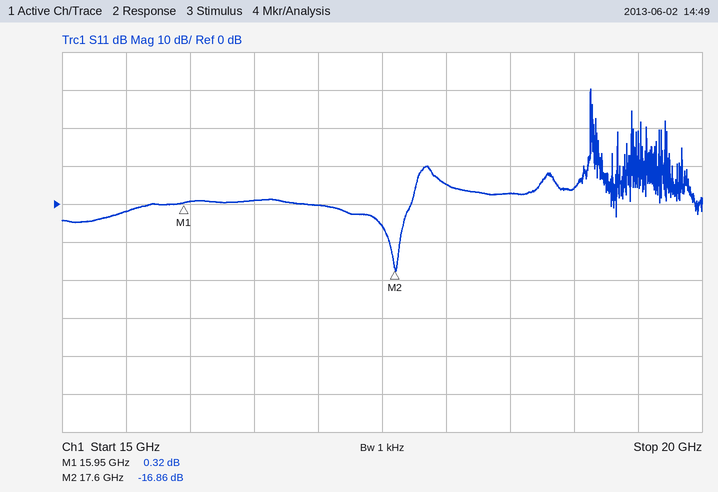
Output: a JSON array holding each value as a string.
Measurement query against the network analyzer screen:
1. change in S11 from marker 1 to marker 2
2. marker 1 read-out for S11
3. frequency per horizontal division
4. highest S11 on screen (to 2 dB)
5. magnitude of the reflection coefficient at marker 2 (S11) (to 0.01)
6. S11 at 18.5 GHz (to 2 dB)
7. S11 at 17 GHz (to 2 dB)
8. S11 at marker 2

["-17.18 dB", "0.32 dB", "500 MHz", "30 dB", "0.14", "2 dB", "0 dB", "-16.86 dB"]
